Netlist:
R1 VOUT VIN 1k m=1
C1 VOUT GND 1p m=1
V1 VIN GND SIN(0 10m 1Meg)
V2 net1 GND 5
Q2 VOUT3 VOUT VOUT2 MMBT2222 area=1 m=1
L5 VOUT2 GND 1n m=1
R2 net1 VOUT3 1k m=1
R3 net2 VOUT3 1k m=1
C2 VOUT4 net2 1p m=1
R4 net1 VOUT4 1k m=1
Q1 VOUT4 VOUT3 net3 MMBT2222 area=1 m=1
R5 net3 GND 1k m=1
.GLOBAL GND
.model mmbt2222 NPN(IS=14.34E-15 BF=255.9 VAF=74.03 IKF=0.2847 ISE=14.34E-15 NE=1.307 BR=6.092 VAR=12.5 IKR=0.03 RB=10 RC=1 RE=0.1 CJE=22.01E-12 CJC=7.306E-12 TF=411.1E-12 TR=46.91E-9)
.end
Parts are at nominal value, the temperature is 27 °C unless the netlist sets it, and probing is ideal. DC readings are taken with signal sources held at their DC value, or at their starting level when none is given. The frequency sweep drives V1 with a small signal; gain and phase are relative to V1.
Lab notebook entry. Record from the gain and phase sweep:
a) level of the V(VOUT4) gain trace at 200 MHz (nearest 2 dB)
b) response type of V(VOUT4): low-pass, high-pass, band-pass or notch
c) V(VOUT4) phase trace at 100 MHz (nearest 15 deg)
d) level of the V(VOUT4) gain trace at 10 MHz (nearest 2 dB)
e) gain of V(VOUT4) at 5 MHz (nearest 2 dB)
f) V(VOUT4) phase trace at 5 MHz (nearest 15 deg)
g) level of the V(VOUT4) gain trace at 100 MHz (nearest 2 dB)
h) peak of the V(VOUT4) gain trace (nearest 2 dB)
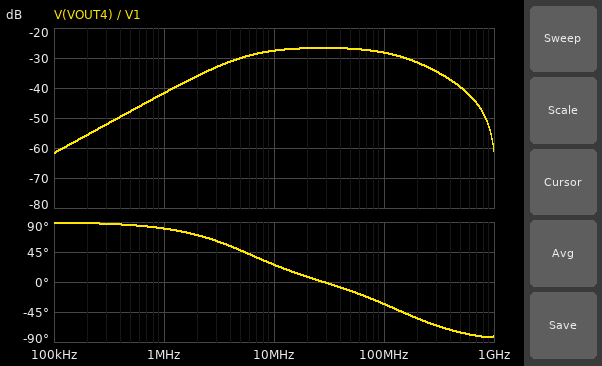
-32 dB
band-pass
-30 deg
-28 dB
-30 dB
45 deg
-28 dB
-26 dB
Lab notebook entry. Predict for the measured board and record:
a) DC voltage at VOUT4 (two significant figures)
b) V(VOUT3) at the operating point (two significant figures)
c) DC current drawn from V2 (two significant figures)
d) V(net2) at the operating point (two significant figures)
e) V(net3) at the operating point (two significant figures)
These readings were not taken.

3.1 V
3.8 V
3.1 mA
3.8 V
3.1 V
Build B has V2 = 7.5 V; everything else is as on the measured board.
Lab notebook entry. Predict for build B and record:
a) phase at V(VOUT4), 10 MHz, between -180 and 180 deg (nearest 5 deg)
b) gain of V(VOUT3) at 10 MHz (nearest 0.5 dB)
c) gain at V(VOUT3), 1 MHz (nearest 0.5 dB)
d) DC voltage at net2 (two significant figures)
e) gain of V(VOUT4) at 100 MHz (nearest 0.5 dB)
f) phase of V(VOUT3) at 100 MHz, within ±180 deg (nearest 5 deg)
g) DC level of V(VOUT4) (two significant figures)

25 deg
-28.0 dB
-42.5 dB
5.5 V
-28.5 dB
-30 deg
4.8 V
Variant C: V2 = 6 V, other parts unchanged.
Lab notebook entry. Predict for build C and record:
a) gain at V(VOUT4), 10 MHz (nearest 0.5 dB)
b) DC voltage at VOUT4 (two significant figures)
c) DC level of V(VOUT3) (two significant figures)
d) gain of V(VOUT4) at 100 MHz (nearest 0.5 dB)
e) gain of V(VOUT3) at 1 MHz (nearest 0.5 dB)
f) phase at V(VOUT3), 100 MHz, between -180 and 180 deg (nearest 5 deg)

-28.0 dB
3.8 V
4.5 V
-28.5 dB
-42.0 dB
-30 deg
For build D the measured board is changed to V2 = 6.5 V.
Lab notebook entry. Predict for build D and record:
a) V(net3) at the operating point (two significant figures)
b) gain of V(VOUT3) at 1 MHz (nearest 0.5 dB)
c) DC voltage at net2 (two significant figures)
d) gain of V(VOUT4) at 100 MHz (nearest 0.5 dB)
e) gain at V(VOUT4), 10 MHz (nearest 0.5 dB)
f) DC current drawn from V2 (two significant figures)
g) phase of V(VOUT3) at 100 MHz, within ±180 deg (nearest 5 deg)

4.1 V
-42.0 dB
4.8 V
-28.5 dB
-28.0 dB
4.1 mA
-30 deg
